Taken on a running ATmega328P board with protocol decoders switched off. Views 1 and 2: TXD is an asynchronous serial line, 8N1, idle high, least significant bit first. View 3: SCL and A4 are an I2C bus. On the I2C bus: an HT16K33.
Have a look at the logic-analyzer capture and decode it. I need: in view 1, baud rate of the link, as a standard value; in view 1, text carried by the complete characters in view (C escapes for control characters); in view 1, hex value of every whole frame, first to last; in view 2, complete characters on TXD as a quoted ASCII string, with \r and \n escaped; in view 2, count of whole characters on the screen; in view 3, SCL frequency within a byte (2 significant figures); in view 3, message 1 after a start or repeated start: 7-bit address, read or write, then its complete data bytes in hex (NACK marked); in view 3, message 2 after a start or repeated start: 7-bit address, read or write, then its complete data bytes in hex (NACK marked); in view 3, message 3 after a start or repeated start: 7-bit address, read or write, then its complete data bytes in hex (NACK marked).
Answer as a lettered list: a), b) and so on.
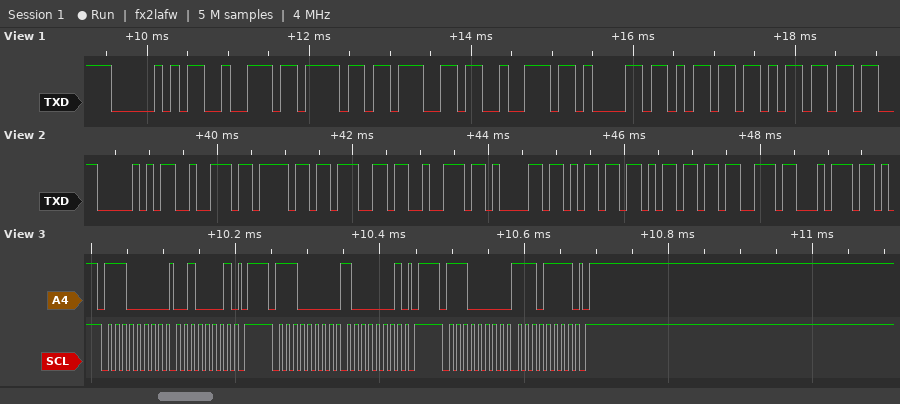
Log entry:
a) 9600 baud
b) "Programm"
c) 0x50 0x72 0x6F 0x67 0x72 0x61 0x6D 0x6D
d) "Programmst"
e) 10
f) 100 kHz
g) 0x70 write: 21
h) 0x70 write: 81
i) 0x70 write: EF
